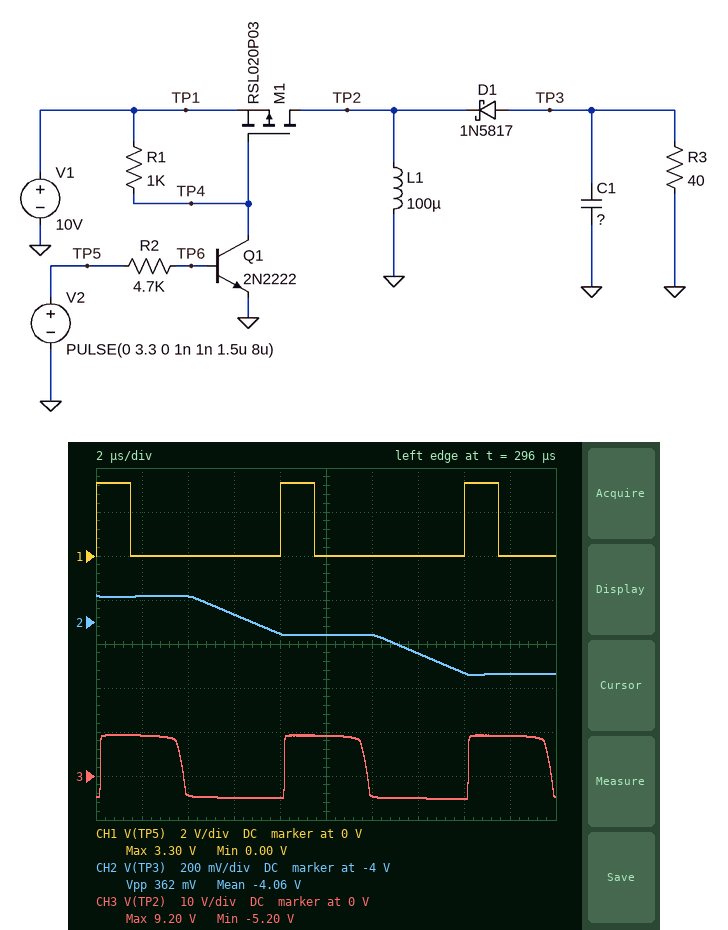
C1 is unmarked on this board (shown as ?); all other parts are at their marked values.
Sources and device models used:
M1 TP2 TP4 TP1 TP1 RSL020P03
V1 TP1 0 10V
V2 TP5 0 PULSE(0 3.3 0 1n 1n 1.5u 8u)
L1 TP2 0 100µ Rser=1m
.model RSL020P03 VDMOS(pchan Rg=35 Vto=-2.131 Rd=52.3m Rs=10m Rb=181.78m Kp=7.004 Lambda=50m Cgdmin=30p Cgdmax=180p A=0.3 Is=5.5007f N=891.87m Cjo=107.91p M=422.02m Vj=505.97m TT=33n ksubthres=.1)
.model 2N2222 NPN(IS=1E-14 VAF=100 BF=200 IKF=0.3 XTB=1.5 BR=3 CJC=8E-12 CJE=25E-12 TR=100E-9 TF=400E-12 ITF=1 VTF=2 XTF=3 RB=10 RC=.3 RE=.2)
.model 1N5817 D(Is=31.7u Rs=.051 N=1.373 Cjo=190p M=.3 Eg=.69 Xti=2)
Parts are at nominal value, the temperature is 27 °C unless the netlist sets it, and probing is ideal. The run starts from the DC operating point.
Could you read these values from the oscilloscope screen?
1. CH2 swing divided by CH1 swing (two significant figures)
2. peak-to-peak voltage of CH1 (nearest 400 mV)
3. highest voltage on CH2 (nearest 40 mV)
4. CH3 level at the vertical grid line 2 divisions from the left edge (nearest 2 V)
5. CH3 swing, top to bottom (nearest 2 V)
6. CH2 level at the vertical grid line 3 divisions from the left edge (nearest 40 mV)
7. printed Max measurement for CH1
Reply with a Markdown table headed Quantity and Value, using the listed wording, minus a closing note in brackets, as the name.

| Quantity | Value |
|---|---|
| CH2 swing divided by CH1 swing | 0.11 |
| peak-to-peak voltage of CH1 | 3.2 V |
| highest voltage on CH2 | -3.88 V |
| CH3 level at the vertical grid line 2 divisions from the left edge | -4 V |
| CH3 swing, top to bottom | 14 V |
| CH2 level at the vertical grid line 3 divisions from the left edge | -3.96 V |
| printed Max measurement for CH1 | 3.30 V |
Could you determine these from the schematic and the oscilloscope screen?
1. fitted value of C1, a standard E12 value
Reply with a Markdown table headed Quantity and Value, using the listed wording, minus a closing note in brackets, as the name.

| Quantity | Value |
|---|---|
| fitted value of C1, a standard E12 value | 220 µF |
